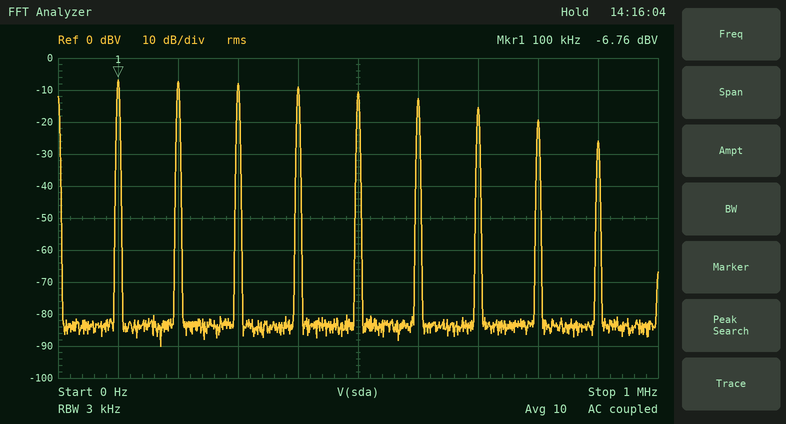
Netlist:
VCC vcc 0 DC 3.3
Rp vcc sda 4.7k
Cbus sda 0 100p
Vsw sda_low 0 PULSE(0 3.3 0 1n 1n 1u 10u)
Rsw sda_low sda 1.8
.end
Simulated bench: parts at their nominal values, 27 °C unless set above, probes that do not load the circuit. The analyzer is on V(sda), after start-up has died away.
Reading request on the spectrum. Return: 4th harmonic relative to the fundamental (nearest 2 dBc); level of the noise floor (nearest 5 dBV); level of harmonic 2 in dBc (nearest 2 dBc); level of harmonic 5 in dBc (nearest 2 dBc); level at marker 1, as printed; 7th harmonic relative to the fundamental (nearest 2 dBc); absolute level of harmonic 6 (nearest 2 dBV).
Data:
-2 dBc
-85 dBV
0 dBc
-4 dBc
-6.76 dBV
-8 dBc
-12 dBV
